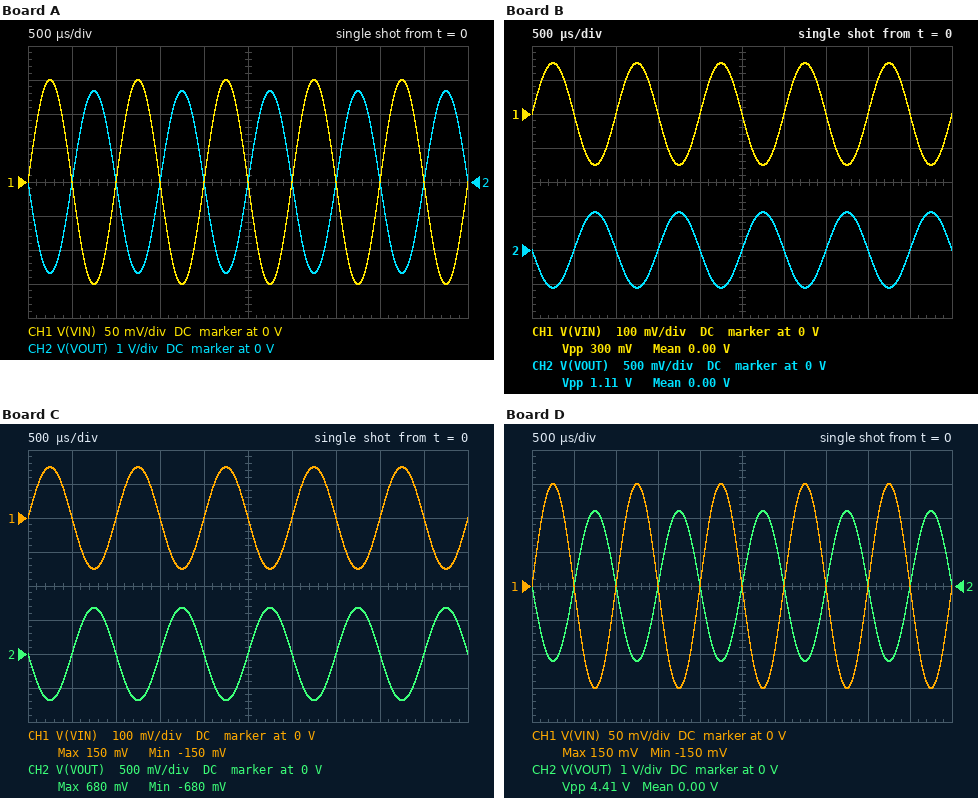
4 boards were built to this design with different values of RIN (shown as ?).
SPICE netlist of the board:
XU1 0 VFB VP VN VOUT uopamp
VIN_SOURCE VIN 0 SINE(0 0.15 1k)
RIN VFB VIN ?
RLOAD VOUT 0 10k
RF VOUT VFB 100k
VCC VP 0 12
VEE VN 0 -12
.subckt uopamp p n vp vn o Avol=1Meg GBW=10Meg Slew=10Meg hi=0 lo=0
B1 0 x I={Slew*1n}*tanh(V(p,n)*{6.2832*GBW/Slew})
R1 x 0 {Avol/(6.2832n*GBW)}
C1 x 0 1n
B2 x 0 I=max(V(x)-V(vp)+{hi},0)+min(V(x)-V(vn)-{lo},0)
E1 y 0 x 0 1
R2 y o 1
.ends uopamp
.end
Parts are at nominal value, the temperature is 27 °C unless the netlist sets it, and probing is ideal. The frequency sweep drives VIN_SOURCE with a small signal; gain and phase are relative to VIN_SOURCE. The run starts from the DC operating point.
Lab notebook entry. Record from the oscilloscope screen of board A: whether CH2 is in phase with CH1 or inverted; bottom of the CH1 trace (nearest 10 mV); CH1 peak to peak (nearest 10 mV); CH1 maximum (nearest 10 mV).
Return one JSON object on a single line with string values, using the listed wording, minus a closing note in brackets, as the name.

{"whether CH2 is in phase with CH1 or inverted": "inverted", "bottom of the CH1 trace": "-150 mV", "CH1 peak to peak": "300 mV", "CH1 maximum": "150 mV"}
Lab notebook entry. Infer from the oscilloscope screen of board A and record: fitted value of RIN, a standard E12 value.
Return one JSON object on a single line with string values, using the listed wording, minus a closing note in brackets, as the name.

{"fitted value of RIN, a standard E12 value": "5.6 kΩ"}
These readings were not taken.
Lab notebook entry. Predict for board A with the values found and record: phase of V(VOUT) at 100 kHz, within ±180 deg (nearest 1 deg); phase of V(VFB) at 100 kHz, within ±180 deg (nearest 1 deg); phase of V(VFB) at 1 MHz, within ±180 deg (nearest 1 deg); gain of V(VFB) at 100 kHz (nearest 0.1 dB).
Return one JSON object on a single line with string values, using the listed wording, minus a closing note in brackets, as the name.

{"phase of V(VOUT) at 100 kHz, within ±180 deg": "169 deg", "phase of V(VFB) at 100 kHz, within ±180 deg": "79 deg", "phase of V(VFB) at 1 MHz, within ±180 deg": "28 deg", "gain of V(VFB) at 100 kHz": "-15.1 dB"}
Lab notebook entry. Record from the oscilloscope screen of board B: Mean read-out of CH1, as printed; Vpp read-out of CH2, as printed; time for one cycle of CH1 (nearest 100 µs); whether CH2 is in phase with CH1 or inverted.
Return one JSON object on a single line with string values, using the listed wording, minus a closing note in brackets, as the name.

{"Mean read-out of CH1, as printed": "0.00 V", "Vpp read-out of CH2, as printed": "1.11 V", "time for one cycle of CH1": "1.0 ms", "whether CH2 is in phase with CH1 or inverted": "inverted"}
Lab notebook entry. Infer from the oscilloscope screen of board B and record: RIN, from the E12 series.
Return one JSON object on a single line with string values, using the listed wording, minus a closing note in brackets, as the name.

{"RIN, from the E12 series": "27 kΩ"}
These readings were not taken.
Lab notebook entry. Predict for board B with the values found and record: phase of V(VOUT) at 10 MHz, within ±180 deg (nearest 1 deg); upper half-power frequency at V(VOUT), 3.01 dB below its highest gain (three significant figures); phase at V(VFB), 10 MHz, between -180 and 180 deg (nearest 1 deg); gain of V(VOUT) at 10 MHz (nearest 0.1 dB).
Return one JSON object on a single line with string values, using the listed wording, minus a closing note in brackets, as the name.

{"phase of V(VOUT) at 10 MHz, within ±180 deg": "102 deg", "upper half-power frequency at V(VOUT), 3.01 dB below its highest gain": "2.13 MHz", "phase at V(VFB), 10 MHz, between -180 and 180 deg": "12 deg", "gain of V(VOUT) at 10 MHz": "-2.3 dB"}
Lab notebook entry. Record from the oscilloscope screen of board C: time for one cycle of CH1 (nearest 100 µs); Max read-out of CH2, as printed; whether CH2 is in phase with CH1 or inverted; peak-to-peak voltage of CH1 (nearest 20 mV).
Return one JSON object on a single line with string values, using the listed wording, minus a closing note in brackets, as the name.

{"time for one cycle of CH1": "1.0 ms", "Max read-out of CH2, as printed": "680 mV", "whether CH2 is in phase with CH1 or inverted": "inverted", "peak-to-peak voltage of CH1": "300 mV"}
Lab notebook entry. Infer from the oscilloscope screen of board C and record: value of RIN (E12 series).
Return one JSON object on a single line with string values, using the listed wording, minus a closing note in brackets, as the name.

{"value of RIN": "22 kΩ"}
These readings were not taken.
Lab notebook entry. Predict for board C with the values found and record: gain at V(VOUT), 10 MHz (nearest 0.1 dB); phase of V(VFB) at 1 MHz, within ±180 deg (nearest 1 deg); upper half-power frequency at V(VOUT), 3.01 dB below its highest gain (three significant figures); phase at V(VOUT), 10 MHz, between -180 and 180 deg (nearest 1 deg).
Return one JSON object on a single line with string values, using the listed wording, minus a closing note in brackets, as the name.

{"gain at V(VOUT), 10 MHz": "-1.9 dB", "phase of V(VFB) at 1 MHz, within ±180 deg": "61 deg", "upper half-power frequency at V(VOUT), 3.01 dB below its highest gain": "1.80 MHz", "phase at V(VOUT), 10 MHz, between -180 and 180 deg": "100 deg"}
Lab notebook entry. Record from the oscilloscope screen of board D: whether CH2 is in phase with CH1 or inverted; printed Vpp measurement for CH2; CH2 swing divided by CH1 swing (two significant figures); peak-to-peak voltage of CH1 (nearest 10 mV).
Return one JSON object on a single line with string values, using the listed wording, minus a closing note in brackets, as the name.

{"whether CH2 is in phase with CH1 or inverted": "inverted", "printed Vpp measurement for CH2": "4.41 V", "CH2 swing divided by CH1 swing": "15", "peak-to-peak voltage of CH1": "300 mV"}
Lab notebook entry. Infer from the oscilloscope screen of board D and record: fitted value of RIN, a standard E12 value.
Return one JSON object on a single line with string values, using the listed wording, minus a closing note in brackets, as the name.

{"fitted value of RIN, a standard E12 value": "6.8 kΩ"}
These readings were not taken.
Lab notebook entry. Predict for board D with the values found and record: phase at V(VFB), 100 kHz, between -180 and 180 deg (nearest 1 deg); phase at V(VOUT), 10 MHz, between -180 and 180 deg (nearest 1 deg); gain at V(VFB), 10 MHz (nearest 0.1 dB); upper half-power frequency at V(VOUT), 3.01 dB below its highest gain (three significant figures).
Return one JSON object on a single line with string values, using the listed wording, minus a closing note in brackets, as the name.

{"phase at V(VFB), 100 kHz, between -180 and 180 deg": "81 deg", "phase at V(VOUT), 10 MHz, between -180 and 180 deg": "94 deg", "gain at V(VFB), 10 MHz": "-0.6 dB", "upper half-power frequency at V(VOUT), 3.01 dB below its highest gain": "637 kHz"}
